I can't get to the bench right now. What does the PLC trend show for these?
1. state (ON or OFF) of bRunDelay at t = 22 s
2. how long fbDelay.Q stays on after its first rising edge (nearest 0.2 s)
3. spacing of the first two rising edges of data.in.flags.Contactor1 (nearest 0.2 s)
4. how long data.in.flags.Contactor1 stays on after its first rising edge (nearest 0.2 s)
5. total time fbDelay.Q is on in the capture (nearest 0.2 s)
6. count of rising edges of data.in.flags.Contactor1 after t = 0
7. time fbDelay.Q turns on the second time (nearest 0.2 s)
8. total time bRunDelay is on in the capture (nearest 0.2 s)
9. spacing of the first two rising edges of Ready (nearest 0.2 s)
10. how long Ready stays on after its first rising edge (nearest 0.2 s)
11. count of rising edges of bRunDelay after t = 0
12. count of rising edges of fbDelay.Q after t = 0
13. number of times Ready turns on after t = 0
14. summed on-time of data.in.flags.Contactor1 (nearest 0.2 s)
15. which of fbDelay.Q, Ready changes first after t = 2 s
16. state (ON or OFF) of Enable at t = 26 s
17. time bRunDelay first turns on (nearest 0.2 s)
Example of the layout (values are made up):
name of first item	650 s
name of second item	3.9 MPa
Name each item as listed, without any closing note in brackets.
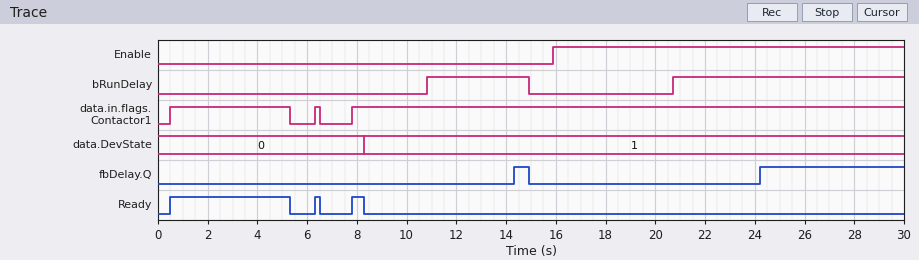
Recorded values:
state (ON or OFF) of bRunDelay at t = 22 s	ON
how long fbDelay.Q stays on after its first rising edge	0.6 s
spacing of the first two rising edges of data.in.flags.Contactor1	5.8 s
how long data.in.flags.Contactor1 stays on after its first rising edge	4.8 s
total time fbDelay.Q is on in the capture	6.4 s
count of rising edges of data.in.flags.Contactor1 after t = 0	3
time fbDelay.Q turns on the second time	24.2 s
total time bRunDelay is on in the capture	13.4 s
spacing of the first two rising edges of Ready	5.8 s
how long Ready stays on after its first rising edge	4.8 s
count of rising edges of bRunDelay after t = 0	2
count of rising edges of fbDelay.Q after t = 0	2
number of times Ready turns on after t = 0	3
summed on-time of data.in.flags.Contactor1	27.2 s
which of fbDelay.Q, Ready changes first after t = 2 s	Ready
state (ON or OFF) of Enable at t = 26 s	ON
time bRunDelay first turns on	10.8 s
